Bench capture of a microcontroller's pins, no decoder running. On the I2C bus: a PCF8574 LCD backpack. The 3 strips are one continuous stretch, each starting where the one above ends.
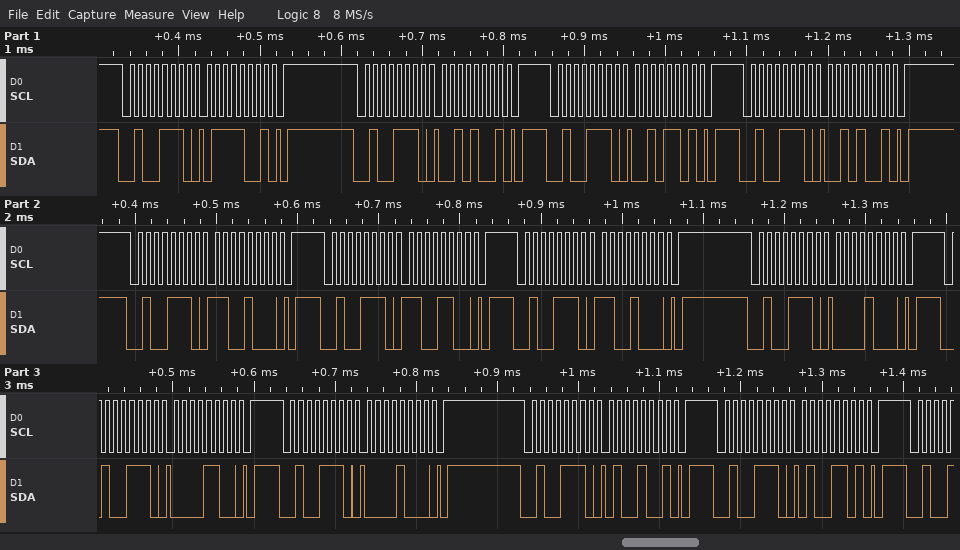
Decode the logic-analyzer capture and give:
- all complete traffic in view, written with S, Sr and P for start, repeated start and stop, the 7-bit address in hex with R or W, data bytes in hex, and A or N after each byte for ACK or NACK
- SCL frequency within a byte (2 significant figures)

S 27W A 79 A P S 27W A 29 A P S 27W A 2D A P S 27W A 29 A P S 27W A C8 A P S 27W A CC A P S 27W A C8 A P S 27W A 08 A P S 27W A 0C A P S 27W A 08 A P S 27W A 49 A P S 27W A 4D A P
100 kHz
